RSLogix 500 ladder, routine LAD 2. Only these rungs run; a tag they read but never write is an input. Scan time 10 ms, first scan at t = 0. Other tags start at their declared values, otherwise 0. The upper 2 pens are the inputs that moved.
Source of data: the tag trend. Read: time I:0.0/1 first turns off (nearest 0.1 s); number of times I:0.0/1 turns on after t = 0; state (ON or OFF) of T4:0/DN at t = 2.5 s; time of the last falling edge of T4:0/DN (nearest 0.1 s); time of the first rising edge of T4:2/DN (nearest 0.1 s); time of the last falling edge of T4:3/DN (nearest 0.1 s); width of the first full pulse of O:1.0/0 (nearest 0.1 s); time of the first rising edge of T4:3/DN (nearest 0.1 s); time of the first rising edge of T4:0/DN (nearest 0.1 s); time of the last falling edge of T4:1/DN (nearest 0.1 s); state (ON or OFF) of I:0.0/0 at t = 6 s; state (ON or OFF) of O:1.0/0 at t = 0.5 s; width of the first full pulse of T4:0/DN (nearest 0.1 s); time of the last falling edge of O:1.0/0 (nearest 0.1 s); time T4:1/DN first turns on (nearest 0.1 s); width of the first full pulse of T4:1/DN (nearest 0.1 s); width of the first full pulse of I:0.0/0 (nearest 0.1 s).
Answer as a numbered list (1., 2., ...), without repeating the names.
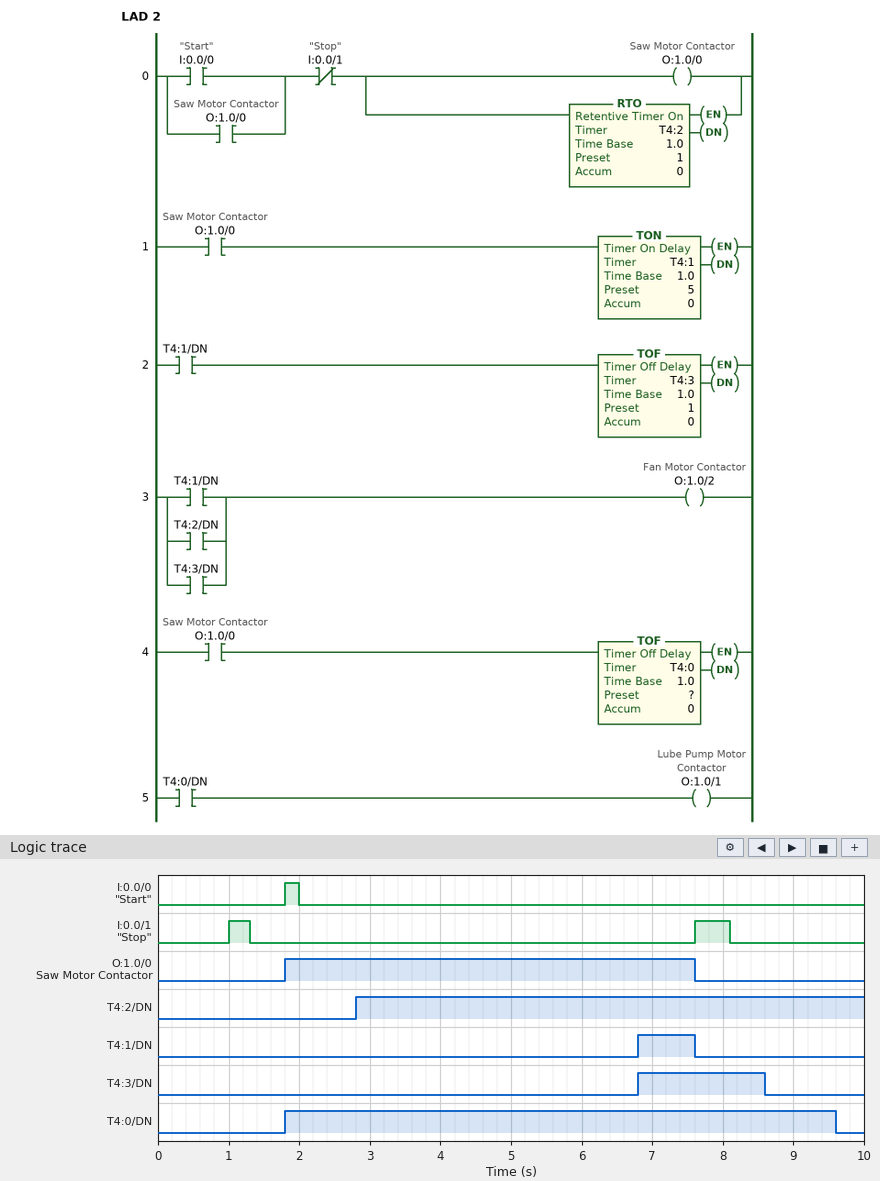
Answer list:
1. 1.3 s
2. 2
3. ON
4. 9.6 s
5. 2.8 s
6. 8.6 s
7. 5.8 s
8. 6.8 s
9. 1.8 s
10. 7.6 s
11. OFF
12. OFF
13. 7.8 s
14. 7.6 s
15. 6.8 s
16. 0.8 s
17. 0.2 s
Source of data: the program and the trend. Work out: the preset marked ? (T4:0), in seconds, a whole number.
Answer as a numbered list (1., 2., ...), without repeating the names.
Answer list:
1. 2 s
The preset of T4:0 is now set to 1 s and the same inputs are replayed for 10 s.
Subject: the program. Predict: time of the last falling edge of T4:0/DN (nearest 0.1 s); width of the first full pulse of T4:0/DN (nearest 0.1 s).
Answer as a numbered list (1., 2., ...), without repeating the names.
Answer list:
1. 8.6 s
2. 6.8 s
